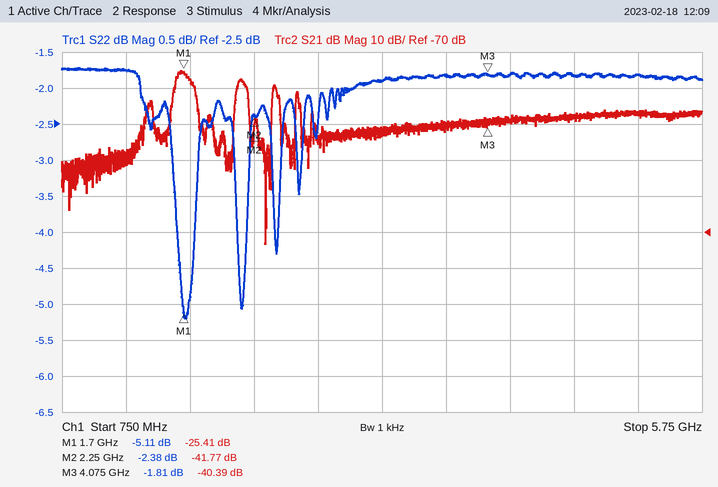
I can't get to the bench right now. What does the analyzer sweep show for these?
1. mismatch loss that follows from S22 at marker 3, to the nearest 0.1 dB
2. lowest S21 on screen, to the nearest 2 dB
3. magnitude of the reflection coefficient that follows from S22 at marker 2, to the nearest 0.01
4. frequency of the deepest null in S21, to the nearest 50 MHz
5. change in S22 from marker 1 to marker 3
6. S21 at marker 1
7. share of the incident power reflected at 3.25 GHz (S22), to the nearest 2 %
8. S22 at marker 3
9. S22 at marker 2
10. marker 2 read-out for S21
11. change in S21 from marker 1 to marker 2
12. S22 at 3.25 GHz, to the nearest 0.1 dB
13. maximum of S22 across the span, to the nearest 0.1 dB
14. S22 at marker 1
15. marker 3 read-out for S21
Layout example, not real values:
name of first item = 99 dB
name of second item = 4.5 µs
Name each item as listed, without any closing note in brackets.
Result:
mismatch loss that follows from S22 at marker 3, to the nearest 0.1 dB = 4.7 dB
lowest S21 on screen, to the nearest 2 dB = -74 dB
magnitude of the reflection coefficient that follows from S22 at marker 2, to the nearest 0.01 = 0.76
frequency of the deepest null in S21, to the nearest 50 MHz = 2.35 GHz
change in S22 from marker 1 to marker 3 = 3.30 dB
S21 at marker 1 = -25.41 dB
share of the incident power reflected at 3.25 GHz (S22), to the nearest 2 % = 64 %
S22 at marker 3 = -1.81 dB
S22 at marker 2 = -2.38 dB
marker 2 read-out for S21 = -41.77 dB
change in S21 from marker 1 to marker 2 = -16.36 dB
S22 at 3.25 GHz, to the nearest 0.1 dB = -1.9 dB
maximum of S22 across the span, to the nearest 0.1 dB = -1.7 dB
S22 at marker 1 = -5.11 dB
marker 3 read-out for S21 = -40.39 dB
